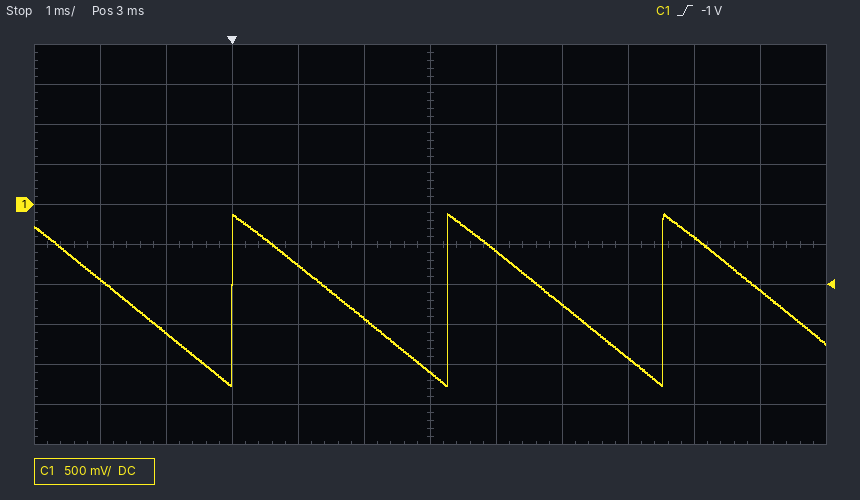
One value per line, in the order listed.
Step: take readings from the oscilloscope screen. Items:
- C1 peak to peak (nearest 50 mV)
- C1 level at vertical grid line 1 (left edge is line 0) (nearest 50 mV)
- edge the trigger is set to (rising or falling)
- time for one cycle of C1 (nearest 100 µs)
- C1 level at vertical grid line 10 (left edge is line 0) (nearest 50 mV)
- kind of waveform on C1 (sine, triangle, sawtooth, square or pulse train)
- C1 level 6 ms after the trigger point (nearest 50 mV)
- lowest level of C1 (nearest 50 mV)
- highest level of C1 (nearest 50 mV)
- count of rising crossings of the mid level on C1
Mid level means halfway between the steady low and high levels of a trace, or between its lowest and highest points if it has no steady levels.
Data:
2.15 V
-950 mV
rising
3.3 ms
-400 mV
sawtooth
-1.90 V
-2.25 V
-100 mV
3
